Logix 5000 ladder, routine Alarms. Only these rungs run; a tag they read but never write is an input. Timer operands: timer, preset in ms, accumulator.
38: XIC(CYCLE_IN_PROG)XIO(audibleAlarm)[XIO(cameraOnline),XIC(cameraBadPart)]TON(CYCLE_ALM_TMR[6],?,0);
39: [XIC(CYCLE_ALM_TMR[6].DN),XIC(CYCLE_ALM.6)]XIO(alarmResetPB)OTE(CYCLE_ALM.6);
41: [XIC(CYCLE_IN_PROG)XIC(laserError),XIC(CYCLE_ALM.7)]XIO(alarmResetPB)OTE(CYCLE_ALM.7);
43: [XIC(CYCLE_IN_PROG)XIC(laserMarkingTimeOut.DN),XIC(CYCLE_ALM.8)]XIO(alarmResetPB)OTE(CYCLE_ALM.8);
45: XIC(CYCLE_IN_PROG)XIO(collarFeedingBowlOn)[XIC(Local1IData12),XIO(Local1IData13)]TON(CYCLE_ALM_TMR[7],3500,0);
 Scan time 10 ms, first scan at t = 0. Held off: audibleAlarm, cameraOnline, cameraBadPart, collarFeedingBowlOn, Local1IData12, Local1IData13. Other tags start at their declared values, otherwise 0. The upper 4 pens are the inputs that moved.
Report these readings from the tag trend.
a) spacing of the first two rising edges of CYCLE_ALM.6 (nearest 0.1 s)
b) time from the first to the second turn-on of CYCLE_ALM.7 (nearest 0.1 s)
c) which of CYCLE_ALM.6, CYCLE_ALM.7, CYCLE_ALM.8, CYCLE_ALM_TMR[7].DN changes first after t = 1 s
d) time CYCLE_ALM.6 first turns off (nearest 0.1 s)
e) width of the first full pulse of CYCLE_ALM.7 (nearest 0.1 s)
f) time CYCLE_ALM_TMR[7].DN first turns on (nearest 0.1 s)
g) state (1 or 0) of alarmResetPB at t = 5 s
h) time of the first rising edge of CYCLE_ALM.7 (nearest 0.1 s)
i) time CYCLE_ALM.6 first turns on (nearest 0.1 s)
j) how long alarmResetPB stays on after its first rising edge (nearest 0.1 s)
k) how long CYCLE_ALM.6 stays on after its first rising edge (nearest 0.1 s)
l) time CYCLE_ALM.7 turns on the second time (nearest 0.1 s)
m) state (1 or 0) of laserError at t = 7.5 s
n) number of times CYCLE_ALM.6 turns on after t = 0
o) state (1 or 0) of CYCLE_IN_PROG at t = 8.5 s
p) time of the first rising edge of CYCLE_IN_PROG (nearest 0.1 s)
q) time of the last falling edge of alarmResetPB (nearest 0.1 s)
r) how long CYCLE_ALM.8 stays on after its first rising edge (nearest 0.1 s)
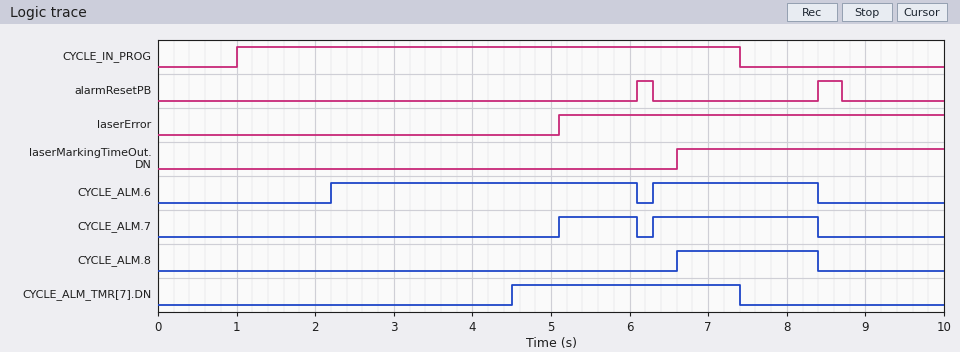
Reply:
4.1 s
1.2 s
CYCLE_ALM.6
6.1 s
1.0 s
4.5 s
0
5.1 s
2.2 s
0.2 s
3.9 s
6.3 s
1
2
0
1.0 s
8.7 s
1.8 s
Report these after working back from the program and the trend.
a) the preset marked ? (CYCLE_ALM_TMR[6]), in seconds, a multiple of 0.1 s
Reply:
1.2 s
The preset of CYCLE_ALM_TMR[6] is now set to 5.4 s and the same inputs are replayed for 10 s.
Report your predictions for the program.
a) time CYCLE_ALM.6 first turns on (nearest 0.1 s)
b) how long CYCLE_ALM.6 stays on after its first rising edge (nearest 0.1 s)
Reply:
6.4 s
2.0 s
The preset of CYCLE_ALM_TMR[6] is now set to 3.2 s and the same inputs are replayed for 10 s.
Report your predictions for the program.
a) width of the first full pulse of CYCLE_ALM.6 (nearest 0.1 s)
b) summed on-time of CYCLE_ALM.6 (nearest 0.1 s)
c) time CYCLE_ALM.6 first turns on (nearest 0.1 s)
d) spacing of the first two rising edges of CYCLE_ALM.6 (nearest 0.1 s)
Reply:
1.9 s
4.0 s
4.2 s
2.1 s
